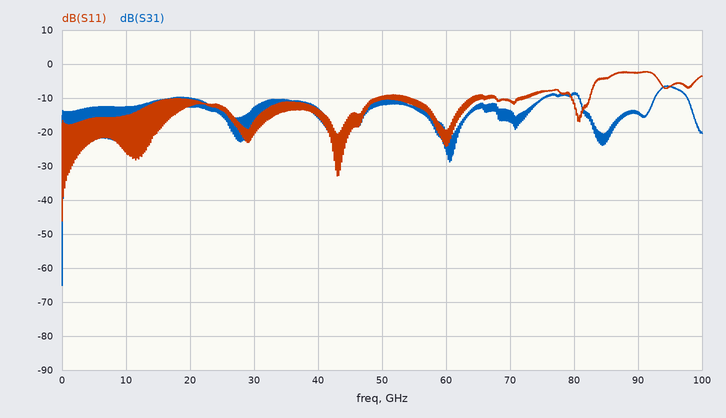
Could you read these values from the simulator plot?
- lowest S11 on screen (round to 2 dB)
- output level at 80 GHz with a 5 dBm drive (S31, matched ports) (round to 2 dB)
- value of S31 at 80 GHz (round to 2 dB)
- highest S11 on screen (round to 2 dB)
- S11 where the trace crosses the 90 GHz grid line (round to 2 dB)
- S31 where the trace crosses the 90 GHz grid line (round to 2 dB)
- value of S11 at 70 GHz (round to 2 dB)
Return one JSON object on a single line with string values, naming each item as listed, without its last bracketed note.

{"lowest S11 on screen": "-46 dB", "output level at 80 GHz with a 5 dBm drive (S31, matched ports)": "-4 dBm", "value of S31 at 80 GHz": "-8 dB", "highest S11 on screen": "-2 dB", "S11 where the trace crosses the 90 GHz grid line": "-2 dB", "S31 where the trace crosses the 90 GHz grid line": "-14 dB", "value of S11 at 70 GHz": "-10 dB"}
